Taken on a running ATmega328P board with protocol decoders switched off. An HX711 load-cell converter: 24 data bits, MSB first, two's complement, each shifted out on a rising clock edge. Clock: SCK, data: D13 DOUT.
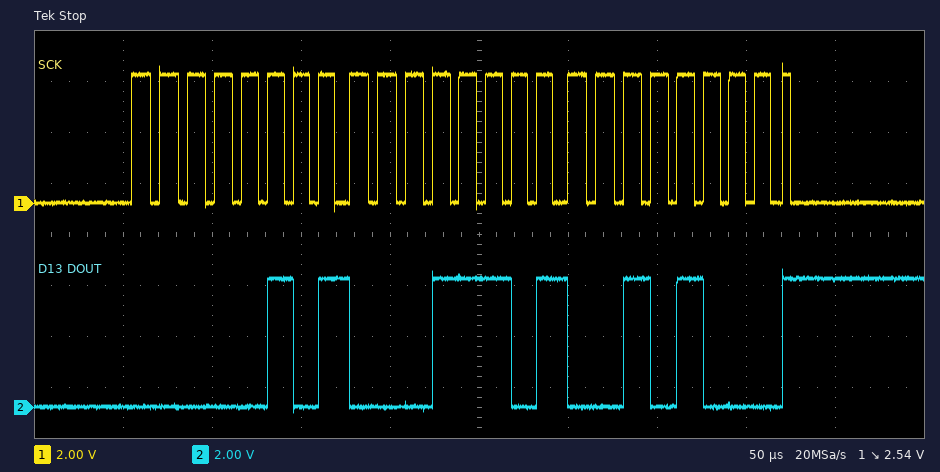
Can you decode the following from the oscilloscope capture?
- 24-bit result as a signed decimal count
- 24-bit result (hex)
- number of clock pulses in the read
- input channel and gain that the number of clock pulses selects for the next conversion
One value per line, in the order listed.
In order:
335144
0x051D28
25
channel A, gain 128
